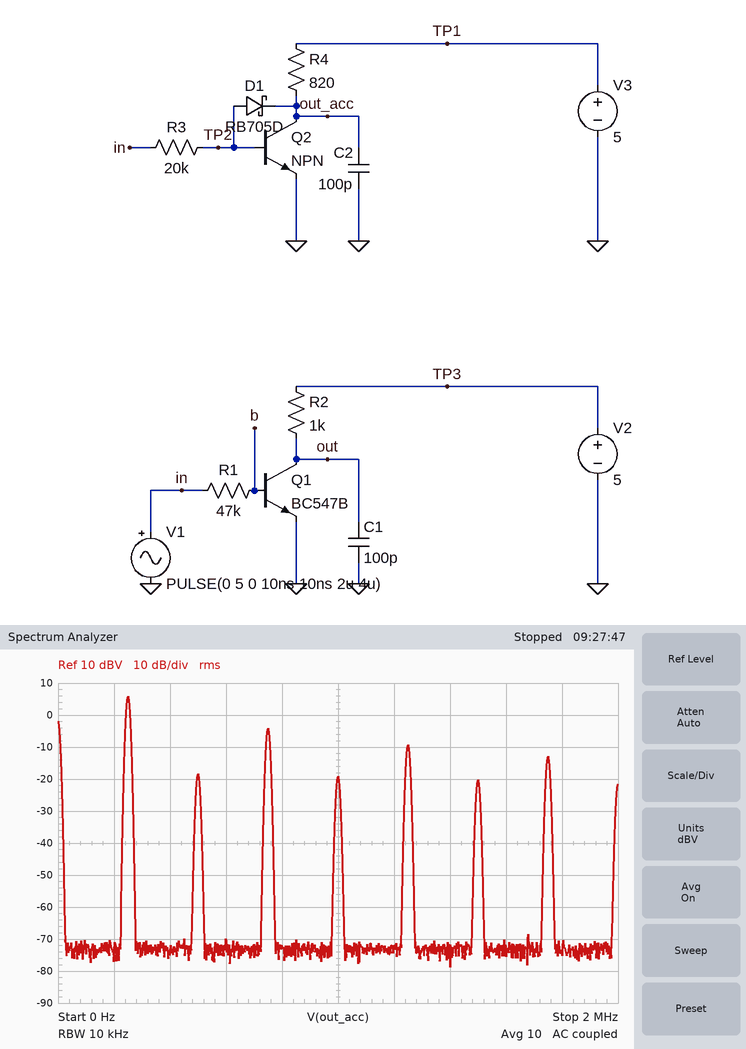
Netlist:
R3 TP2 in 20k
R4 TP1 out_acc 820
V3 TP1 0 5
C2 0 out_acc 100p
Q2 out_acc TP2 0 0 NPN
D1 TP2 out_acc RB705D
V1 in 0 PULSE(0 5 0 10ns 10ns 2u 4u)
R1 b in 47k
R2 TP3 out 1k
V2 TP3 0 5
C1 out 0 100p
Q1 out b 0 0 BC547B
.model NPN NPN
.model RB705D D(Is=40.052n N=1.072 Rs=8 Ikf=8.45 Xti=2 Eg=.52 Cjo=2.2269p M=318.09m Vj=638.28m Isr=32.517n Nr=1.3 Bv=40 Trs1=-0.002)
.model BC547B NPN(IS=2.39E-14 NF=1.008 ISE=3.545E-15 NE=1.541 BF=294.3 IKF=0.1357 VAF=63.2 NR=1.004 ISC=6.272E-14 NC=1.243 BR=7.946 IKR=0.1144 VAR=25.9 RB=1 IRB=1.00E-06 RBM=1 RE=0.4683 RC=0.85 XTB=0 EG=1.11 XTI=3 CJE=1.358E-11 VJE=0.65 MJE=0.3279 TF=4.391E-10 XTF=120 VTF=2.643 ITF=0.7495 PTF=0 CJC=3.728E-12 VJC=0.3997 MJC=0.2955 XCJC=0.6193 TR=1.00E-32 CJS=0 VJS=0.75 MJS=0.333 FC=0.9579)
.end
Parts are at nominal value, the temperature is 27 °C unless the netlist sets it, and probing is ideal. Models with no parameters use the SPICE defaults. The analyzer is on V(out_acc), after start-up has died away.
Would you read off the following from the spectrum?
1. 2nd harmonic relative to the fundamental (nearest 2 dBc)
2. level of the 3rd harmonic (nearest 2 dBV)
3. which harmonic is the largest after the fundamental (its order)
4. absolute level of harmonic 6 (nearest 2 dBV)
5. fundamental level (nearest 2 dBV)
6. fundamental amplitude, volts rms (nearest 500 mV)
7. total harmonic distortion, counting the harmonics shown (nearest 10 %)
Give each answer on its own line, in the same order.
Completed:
-24 dBc
-4 dBV
3
-20 dBV
6 dBV
2.0 V
40 %
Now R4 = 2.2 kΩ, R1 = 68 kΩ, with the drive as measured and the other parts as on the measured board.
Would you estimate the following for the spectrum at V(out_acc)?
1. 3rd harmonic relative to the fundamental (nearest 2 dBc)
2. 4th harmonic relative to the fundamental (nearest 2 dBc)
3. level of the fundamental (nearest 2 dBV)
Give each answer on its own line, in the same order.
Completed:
-12 dBc
-20 dBc
6 dBV
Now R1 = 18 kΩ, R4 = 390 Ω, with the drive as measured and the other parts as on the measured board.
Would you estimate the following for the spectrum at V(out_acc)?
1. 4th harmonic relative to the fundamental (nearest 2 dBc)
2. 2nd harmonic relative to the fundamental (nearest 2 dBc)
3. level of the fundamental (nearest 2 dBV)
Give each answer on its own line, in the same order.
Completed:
-32 dBc
-32 dBc
6 dBV
